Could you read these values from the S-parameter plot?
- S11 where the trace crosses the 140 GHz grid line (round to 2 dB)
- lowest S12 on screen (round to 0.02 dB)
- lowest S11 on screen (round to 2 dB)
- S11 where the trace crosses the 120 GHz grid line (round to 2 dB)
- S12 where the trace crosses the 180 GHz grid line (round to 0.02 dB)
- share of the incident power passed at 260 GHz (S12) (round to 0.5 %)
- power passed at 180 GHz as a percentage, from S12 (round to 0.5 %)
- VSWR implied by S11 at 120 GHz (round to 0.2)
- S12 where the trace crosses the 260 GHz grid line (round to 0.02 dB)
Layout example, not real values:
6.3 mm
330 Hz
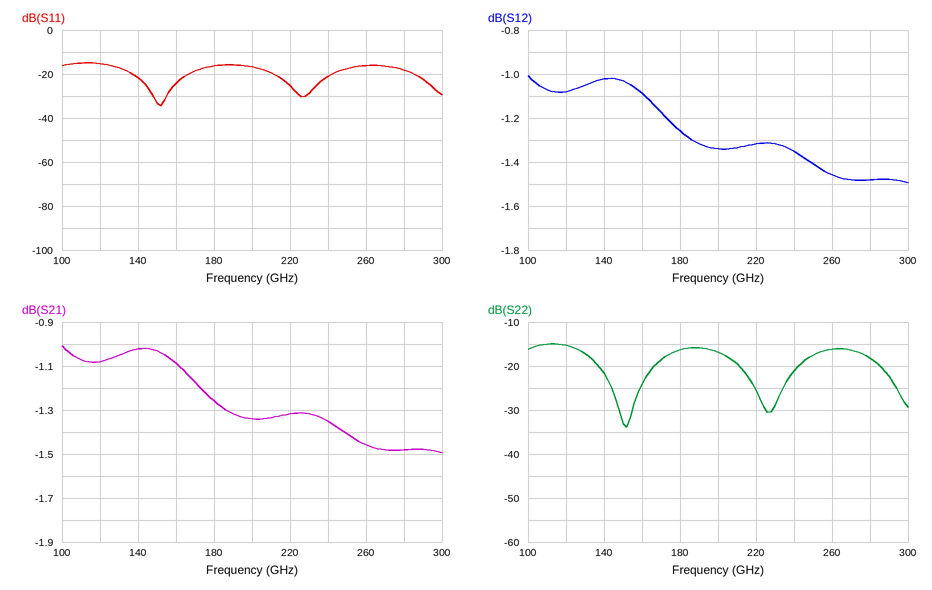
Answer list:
-22 dB
-1.50 dB
-34 dB
-16 dB
-1.26 dB
71.5 %
75.0 %
1.4
-1.46 dB
